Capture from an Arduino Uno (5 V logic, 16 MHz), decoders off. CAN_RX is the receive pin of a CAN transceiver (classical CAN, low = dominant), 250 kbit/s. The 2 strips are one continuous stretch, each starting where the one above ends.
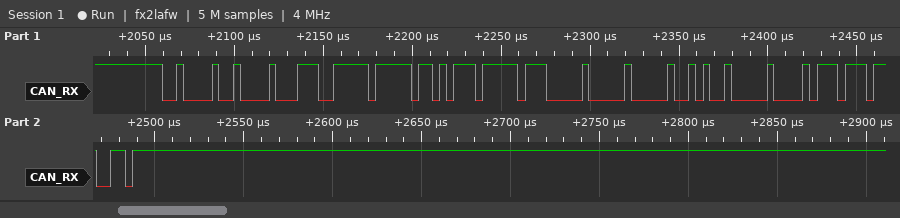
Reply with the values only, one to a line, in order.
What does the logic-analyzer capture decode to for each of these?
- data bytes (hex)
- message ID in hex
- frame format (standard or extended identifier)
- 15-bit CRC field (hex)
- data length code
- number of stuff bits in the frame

E7 FF AE FF 00 00 52 00
0x212
standard
0x5DD9
8
7
